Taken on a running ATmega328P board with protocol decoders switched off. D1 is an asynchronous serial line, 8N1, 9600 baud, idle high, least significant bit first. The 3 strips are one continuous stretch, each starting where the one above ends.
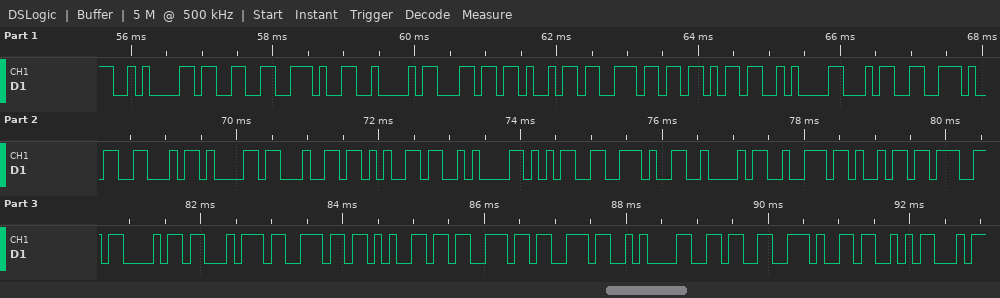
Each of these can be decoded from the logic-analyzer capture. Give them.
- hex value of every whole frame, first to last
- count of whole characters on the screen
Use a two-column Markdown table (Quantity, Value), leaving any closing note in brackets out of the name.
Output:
| Quantity | Value |
|---|---|
| hex value of every whole frame, first to last | 0A 33 2E 42 6C 69 6E 6B 0A 34 2E 46 61 64 65 0A 35 2E 42 72 69 67 68 74 6E 65 73 73 0A 36 2E 53 |
| count of whole characters on the screen | 32 |
